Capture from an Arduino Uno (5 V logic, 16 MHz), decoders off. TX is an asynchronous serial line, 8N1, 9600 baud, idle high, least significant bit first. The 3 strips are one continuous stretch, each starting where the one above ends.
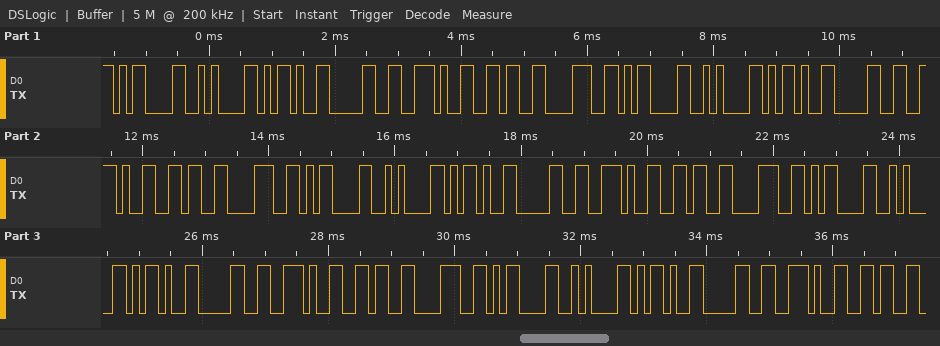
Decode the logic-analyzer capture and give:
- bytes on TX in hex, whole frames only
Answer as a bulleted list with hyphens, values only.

- 0D 0A 2D 30 2E 36 38 0D 0A 2D 30 2E 36 38 0D 0A 2D 30 2E 36 38 0D 0A 2D 30 2E 36 38 0D 0A 2D 30 2E 36
